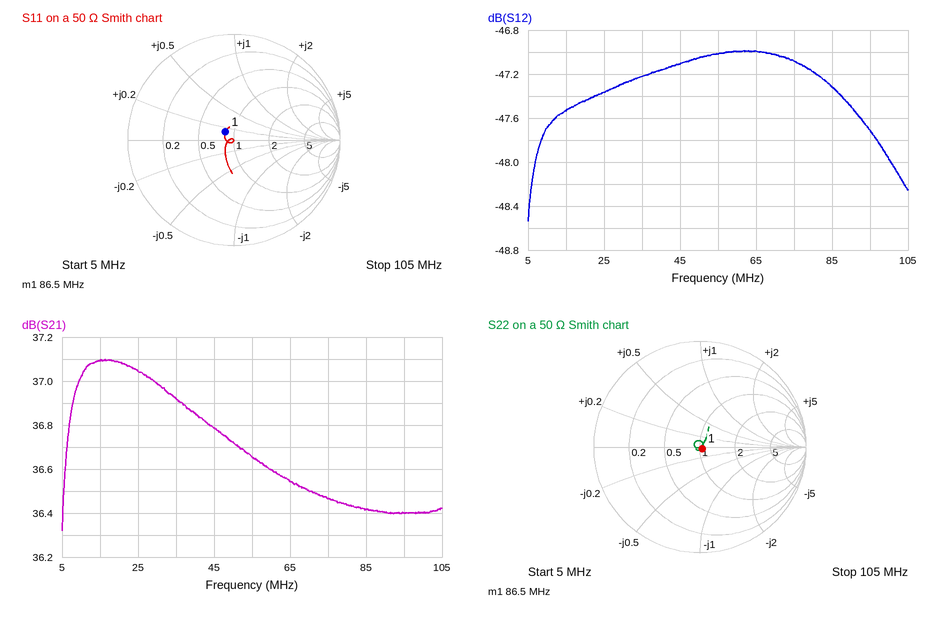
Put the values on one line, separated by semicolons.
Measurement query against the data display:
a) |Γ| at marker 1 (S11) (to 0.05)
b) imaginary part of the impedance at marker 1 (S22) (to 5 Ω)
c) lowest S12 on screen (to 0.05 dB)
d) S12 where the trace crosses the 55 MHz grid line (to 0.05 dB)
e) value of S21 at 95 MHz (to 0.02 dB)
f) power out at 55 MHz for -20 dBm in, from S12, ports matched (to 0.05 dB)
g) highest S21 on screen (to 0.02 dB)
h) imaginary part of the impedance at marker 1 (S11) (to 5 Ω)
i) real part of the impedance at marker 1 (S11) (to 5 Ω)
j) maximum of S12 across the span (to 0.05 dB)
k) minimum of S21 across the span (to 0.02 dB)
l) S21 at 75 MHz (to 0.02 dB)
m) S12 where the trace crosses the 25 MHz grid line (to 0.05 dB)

0.10; 0 Ω; -48.55 dB; -47.00 dB; 36.40 dB; -67.00 dBm; 37.10 dB; +5 Ω; 40 Ω; -47.00 dB; 36.32 dB; 36.46 dB; -47.35 dB
